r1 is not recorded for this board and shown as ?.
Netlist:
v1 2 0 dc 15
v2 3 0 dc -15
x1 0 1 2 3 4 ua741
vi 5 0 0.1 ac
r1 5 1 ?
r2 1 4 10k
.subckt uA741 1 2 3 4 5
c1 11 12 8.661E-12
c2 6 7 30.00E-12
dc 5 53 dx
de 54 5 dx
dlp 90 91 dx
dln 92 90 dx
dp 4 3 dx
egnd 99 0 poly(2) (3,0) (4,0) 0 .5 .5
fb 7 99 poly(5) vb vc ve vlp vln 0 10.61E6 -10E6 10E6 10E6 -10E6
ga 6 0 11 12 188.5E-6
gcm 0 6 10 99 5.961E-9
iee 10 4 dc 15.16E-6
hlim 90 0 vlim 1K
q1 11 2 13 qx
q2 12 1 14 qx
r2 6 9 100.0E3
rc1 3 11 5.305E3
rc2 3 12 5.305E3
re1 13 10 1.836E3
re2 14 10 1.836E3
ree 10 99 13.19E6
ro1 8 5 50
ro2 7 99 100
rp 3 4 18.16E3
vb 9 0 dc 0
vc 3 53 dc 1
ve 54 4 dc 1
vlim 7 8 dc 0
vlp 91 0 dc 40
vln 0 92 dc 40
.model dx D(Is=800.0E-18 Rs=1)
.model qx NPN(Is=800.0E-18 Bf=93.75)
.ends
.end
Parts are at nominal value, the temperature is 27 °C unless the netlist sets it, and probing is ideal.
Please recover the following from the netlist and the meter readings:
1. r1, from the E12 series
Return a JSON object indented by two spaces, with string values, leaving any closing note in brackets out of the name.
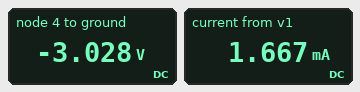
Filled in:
{
  "r1, from the E12 series": "330 Ω"
}
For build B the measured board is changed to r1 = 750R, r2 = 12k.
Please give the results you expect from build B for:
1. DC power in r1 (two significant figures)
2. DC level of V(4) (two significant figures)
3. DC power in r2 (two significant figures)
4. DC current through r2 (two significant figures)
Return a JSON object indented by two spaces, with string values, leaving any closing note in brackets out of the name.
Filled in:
{
  "DC power in r1": "13 µW",
  "DC level of V(4)": "-1.6 V",
  "DC power in r2": "210 µW",
  "DC current through r2": "130 µA"
}
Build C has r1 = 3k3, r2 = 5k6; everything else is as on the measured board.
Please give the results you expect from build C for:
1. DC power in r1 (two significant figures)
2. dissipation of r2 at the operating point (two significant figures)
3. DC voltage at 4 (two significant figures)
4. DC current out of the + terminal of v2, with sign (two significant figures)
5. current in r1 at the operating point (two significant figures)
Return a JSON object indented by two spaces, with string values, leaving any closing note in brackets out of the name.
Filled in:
{
  "DC power in r1": "3.0 µW",
  "dissipation of r2 at the operating point": "5.1 µW",
  "DC voltage at 4": "-170 mV",
  "DC current out of the + terminal of v2, with sign": "-1.7 mA",
  "current in r1 at the operating point": "30 µA"
}
